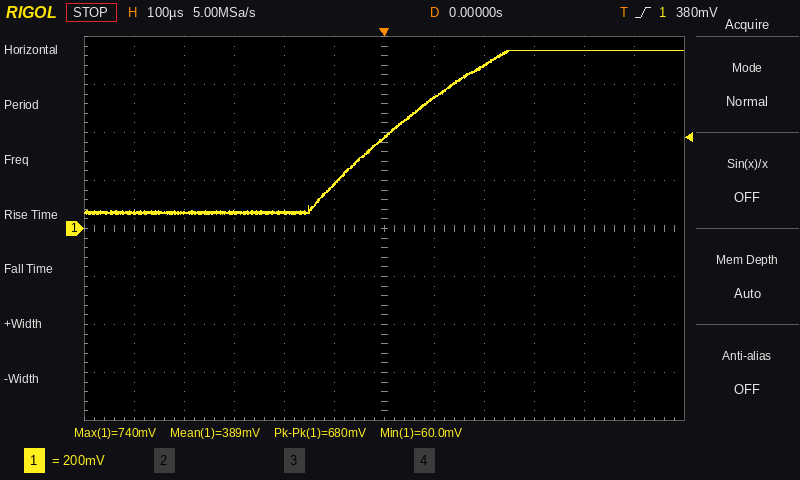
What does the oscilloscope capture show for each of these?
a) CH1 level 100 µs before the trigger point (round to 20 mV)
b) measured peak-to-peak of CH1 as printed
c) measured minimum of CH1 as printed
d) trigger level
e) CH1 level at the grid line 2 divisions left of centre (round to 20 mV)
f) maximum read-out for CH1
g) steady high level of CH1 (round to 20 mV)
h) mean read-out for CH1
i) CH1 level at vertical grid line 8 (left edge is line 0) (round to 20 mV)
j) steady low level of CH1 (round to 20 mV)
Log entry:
180 mV
680 mV
60.0 mV
380 mV
60 mV
740 mV
740 mV
389 mV
680 mV
60 mV
